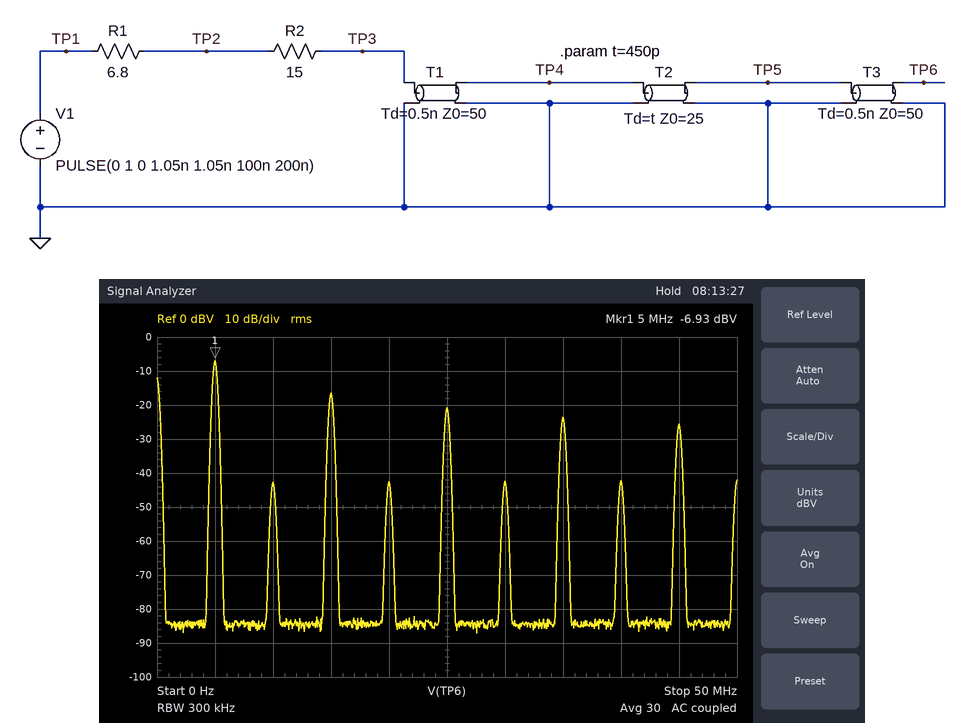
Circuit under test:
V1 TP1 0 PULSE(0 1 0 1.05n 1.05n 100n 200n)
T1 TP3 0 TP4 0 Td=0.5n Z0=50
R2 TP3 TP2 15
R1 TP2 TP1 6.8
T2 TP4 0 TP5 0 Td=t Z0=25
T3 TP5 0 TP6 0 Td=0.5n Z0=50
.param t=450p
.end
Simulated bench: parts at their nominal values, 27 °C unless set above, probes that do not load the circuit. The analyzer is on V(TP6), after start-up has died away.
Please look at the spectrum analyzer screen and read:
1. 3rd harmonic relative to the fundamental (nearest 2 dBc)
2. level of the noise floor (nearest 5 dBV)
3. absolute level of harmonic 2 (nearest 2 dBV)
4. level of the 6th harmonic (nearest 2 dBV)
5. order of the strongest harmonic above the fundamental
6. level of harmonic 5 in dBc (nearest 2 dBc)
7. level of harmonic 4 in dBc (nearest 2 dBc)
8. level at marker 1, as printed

-10 dBc
-85 dBV
-42 dBV
-42 dBV
3
-14 dBc
-36 dBc
-6.93 dBV
